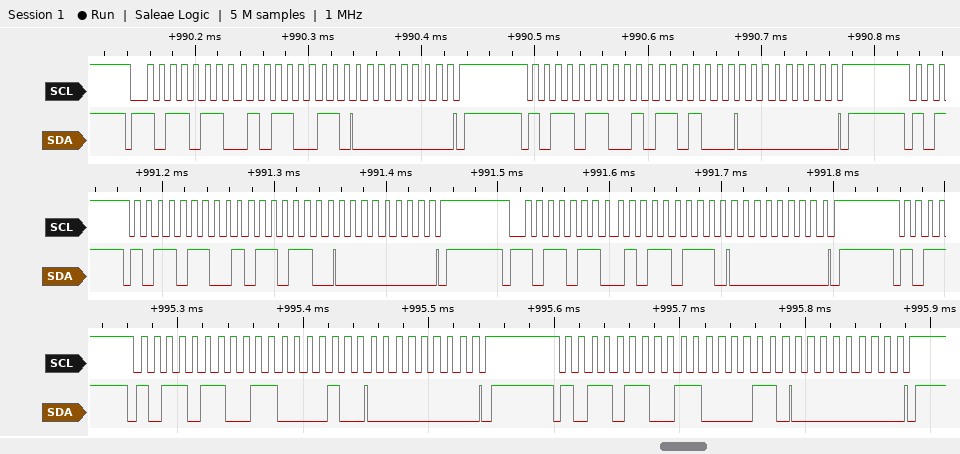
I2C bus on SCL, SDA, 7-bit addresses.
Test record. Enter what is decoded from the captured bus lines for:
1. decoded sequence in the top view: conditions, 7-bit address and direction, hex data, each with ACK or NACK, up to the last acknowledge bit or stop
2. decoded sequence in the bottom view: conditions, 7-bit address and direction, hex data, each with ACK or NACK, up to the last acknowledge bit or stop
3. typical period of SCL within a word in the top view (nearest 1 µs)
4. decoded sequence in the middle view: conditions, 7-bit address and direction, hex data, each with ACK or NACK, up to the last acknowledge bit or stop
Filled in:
start, address 5B write ACK, B3 ACK, 00 ACK, stop, start, address 5B write ACK, B4 ACK, 00 ACK, stop
start, address 5B write ACK, C2 ACK, 00 ACK, stop, start, address 5B write ACK, C3 ACK, 00 ACK, stop
10 µs
start, address 5B write ACK, B6 ACK, 00 ACK, stop, start, address 5B write ACK, B7 ACK, 00 ACK, stop
